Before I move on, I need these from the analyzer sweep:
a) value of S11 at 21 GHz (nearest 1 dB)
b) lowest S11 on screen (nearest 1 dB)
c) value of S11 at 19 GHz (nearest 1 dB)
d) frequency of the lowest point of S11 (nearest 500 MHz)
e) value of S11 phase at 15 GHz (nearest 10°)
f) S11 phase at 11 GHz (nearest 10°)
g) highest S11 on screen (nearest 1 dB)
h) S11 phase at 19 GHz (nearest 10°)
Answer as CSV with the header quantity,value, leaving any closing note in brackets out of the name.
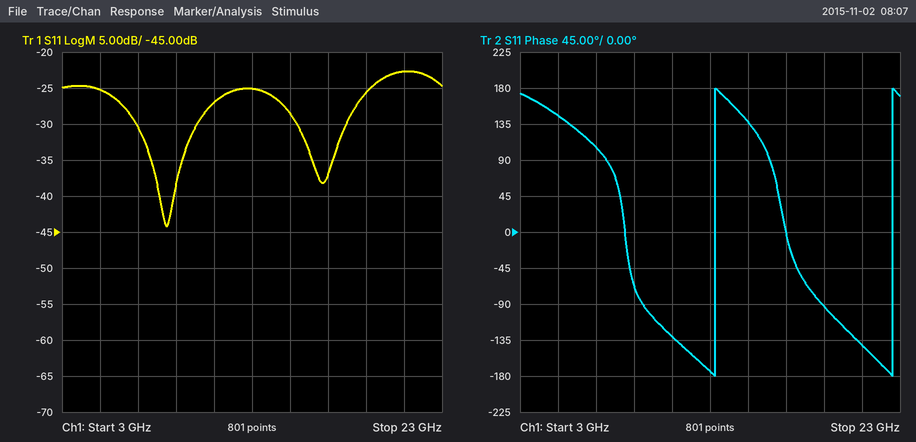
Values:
quantity,value
value of S11 at 21 GHz,-23 dB
lowest S11 on screen,-44 dB
value of S11 at 19 GHz,-26 dB
frequency of the lowest point of S11,8.5 GHz
value of S11 phase at 15 GHz,140°
S11 phase at 11 GHz,-130°
highest S11 on screen,-23 dB
S11 phase at 19 GHz,-90°
